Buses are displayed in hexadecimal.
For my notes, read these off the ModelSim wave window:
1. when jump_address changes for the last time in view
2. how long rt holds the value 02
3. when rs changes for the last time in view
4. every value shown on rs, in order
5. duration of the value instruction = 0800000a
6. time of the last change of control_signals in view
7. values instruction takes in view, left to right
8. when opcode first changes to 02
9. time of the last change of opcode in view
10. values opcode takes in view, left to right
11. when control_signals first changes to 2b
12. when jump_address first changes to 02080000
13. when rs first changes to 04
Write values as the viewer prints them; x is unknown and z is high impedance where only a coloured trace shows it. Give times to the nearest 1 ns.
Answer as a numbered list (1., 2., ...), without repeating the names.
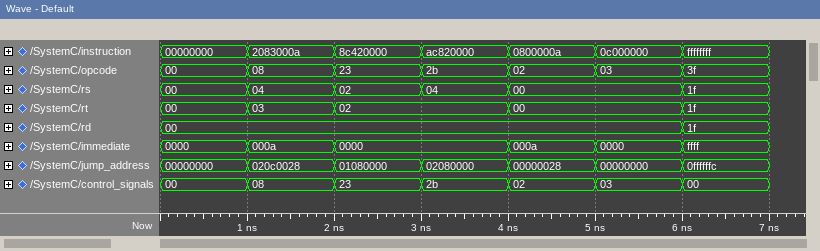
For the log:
1. 6 ns
2. 2 ns
3. 6 ns
4. 00, 04, 02, 04, 00, 1f
5. 1 ns
6. 6 ns
7. 00000000, 2083000a, 8c420000, ac820000, 0800000a, 0c000000, ffffffff
8. 4 ns
9. 6 ns
10. 00, 08, 23, 2b, 02, 03, 3f
11. 3 ns
12. 3 ns
13. 1 ns
